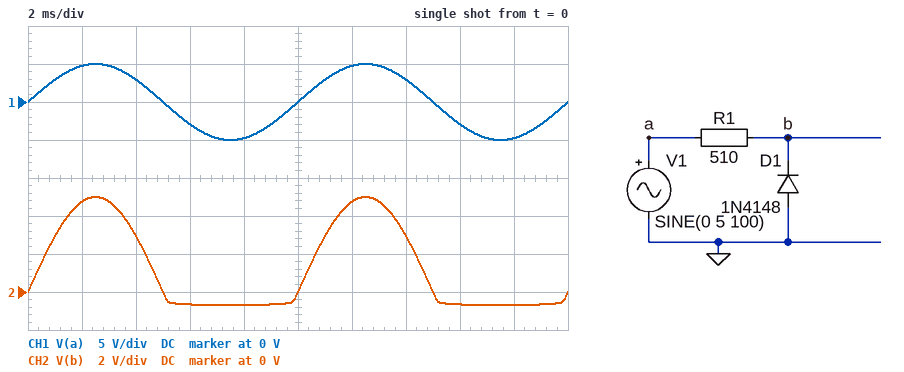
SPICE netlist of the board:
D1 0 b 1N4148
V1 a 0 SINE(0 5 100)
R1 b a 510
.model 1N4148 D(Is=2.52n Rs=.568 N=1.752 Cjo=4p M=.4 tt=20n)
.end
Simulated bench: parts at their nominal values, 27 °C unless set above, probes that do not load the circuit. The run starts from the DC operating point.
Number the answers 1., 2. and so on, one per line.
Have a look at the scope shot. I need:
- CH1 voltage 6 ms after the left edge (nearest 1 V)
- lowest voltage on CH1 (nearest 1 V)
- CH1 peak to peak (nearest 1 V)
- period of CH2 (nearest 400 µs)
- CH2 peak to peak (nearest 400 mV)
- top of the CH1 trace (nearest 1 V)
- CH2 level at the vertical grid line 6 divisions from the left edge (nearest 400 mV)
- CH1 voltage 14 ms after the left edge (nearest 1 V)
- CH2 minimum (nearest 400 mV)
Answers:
1. -3 V
2. -5 V
3. 10 V
4. 10.0 ms
5. 5.6 V
6. 5 V
7. 4.8 V
8. 3 V
9. -800 mV
